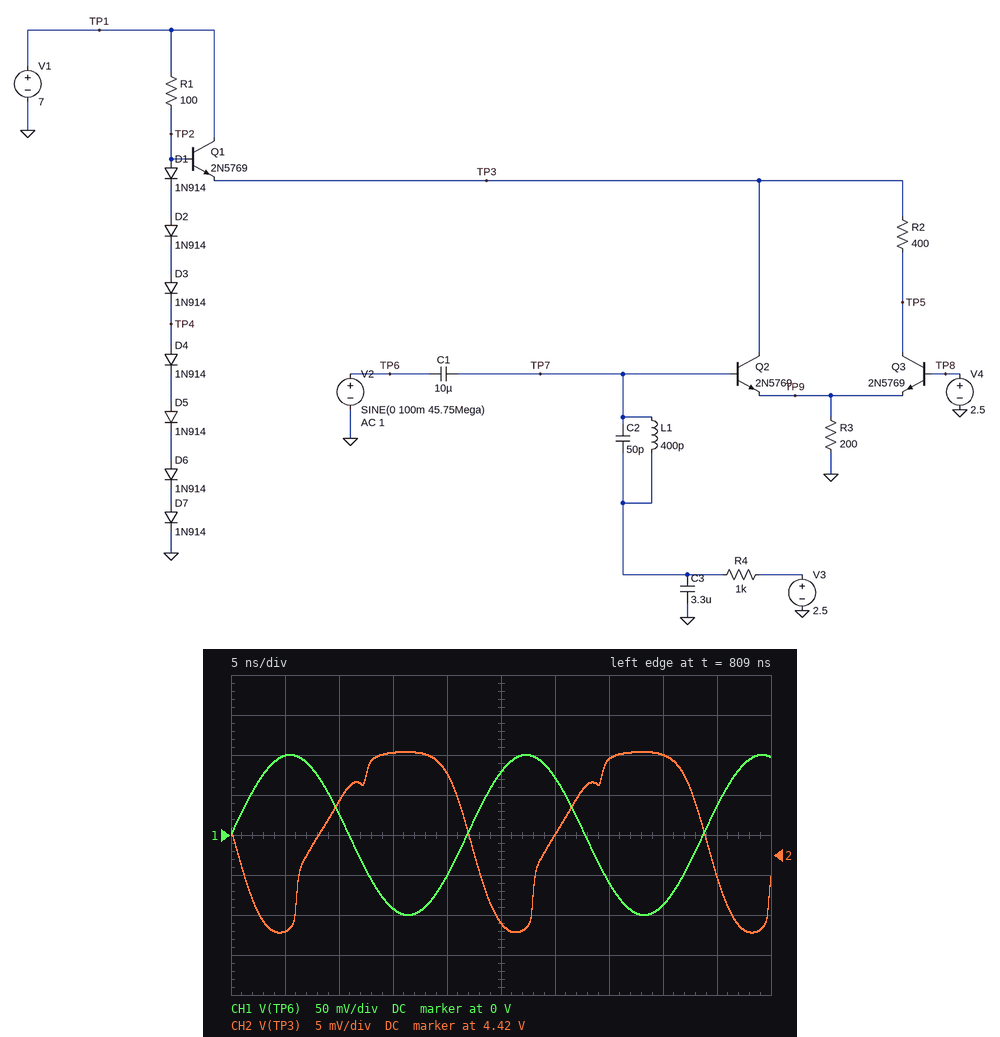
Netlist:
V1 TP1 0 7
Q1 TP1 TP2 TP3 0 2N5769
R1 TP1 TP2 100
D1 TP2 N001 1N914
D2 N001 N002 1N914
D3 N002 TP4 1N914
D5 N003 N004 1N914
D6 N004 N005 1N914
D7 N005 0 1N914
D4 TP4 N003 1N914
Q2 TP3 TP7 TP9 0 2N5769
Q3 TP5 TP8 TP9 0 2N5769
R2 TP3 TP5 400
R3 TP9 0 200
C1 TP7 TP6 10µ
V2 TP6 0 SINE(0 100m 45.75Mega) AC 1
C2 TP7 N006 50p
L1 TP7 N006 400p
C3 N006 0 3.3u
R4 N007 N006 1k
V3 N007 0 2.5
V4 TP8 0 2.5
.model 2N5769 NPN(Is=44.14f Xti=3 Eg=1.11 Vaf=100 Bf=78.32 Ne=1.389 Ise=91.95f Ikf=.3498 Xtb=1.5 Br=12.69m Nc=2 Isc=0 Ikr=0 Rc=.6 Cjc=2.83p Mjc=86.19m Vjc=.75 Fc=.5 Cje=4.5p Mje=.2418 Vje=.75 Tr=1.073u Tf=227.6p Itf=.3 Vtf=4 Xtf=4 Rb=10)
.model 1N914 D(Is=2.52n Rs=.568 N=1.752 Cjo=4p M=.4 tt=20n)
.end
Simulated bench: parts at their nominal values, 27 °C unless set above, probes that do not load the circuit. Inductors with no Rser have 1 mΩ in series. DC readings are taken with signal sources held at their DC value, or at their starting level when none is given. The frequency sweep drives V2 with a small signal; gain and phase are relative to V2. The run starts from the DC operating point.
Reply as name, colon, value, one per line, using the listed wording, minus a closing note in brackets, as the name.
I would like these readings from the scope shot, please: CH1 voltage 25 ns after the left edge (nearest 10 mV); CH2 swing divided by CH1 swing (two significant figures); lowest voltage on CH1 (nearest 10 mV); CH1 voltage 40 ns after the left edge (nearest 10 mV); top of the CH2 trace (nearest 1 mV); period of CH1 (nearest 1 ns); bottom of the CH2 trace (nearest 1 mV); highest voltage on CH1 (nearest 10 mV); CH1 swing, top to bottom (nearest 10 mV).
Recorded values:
CH1 voltage 25 ns after the left edge: 80 mV
CH2 swing divided by CH1 swing: 0.11
lowest voltage on CH1: -100 mV
CH1 voltage 40 ns after the left edge: -90 mV
top of the CH2 trace: 4.433 V
period of CH1: 22 ns
bottom of the CH2 trace: 4.410 V
highest voltage on CH1: 100 mV
CH1 swing, top to bottom: 200 mV
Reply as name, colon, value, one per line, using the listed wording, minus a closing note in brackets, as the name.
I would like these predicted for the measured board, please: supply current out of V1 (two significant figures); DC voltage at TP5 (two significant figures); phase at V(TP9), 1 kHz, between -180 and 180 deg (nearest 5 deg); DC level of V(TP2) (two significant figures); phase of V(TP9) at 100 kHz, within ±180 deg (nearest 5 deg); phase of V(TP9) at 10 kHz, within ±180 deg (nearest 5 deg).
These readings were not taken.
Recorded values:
supply current out of V1: 27 mA
DC voltage at TP5: 2.0 V
phase at V(TP9), 1 kHz, between -180 and 180 deg: 0 deg
DC level of V(TP2): 5.1 V
phase of V(TP9) at 100 kHz, within ±180 deg: 0 deg
phase of V(TP9) at 10 kHz, within ±180 deg: 0 deg
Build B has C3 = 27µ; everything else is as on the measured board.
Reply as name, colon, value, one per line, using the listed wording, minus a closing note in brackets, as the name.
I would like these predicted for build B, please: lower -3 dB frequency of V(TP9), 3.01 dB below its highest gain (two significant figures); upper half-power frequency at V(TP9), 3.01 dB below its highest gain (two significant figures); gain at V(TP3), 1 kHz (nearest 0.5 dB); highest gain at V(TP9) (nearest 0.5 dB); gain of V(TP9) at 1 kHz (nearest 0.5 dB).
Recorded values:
lower -3 dB frequency of V(TP9), 3.01 dB below its highest gain: 2.8 MHz
upper half-power frequency at V(TP9), 3.01 dB below its highest gain: 3.2 MHz
gain at V(TP3), 1 kHz: -29.0 dB
highest gain at V(TP9): 9.0 dB
gain of V(TP9) at 1 kHz: -17.0 dB
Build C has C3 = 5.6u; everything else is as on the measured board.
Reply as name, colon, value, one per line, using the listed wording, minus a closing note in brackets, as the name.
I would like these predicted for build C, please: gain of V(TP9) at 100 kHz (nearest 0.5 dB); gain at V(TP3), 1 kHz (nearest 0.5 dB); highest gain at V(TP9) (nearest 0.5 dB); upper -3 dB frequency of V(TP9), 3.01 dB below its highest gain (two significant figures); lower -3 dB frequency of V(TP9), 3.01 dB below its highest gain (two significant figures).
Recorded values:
gain of V(TP9) at 100 kHz: -9.5 dB
gain at V(TP3), 1 kHz: -21.5 dB
highest gain at V(TP9): 6.5 dB
upper -3 dB frequency of V(TP9), 3.01 dB below its highest gain: 4.5 MHz
lower -3 dB frequency of V(TP9), 3.01 dB below its highest gain: 4.1 MHz
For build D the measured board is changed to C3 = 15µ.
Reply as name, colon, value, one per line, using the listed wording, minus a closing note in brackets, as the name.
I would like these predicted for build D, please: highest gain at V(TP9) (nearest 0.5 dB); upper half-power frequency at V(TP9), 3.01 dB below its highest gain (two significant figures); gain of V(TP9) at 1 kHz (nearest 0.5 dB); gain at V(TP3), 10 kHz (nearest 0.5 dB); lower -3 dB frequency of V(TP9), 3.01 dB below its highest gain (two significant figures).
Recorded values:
highest gain at V(TP9): 8.5 dB
upper half-power frequency at V(TP9), 3.01 dB below its highest gain: 3.5 MHz
gain of V(TP9) at 1 kHz: -13.5 dB
gain at V(TP3), 10 kHz: -25.5 dB
lower -3 dB frequency of V(TP9), 3.01 dB below its highest gain: 3.1 MHz
